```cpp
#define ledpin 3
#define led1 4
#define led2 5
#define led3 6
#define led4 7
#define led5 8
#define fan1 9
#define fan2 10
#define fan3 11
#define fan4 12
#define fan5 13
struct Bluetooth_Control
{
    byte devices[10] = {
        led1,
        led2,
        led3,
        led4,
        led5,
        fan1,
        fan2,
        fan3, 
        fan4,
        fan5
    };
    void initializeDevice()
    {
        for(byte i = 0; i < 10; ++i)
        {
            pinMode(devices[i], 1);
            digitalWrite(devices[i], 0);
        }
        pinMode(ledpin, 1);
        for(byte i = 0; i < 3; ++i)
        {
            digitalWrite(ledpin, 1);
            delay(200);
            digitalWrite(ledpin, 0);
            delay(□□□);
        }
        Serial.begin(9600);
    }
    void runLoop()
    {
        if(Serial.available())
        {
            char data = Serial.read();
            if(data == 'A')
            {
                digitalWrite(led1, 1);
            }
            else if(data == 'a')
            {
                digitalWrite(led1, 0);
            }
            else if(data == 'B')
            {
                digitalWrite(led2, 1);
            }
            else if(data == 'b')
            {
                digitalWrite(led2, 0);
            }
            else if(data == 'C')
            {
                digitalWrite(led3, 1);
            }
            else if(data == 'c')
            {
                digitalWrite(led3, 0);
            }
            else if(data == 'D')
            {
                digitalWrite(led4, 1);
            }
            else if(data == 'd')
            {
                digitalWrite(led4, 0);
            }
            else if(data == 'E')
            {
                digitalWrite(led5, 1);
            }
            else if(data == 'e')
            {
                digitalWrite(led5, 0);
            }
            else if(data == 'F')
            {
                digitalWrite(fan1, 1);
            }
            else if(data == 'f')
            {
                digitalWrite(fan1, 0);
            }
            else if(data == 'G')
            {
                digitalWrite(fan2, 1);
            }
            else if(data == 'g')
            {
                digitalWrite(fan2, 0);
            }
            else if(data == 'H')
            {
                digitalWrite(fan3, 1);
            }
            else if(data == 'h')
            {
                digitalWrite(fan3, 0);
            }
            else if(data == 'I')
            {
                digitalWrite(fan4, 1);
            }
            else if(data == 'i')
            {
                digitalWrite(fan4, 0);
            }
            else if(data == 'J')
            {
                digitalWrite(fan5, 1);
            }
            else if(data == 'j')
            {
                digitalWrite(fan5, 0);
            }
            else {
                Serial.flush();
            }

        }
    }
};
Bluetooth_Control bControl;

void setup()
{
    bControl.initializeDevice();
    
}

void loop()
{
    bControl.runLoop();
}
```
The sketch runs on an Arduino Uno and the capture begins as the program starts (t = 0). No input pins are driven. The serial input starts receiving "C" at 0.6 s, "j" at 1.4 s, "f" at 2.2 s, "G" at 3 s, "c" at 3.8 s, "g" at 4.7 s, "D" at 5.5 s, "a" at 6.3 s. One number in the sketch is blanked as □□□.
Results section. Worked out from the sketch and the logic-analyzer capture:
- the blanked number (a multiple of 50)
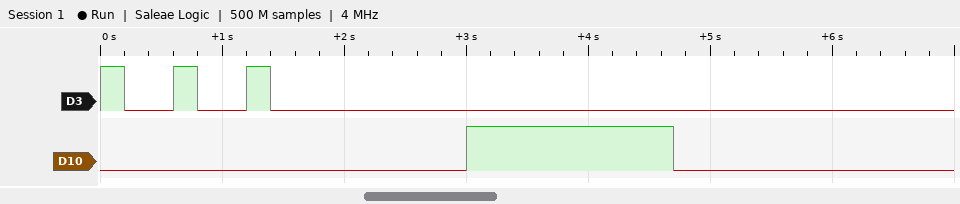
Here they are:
400
